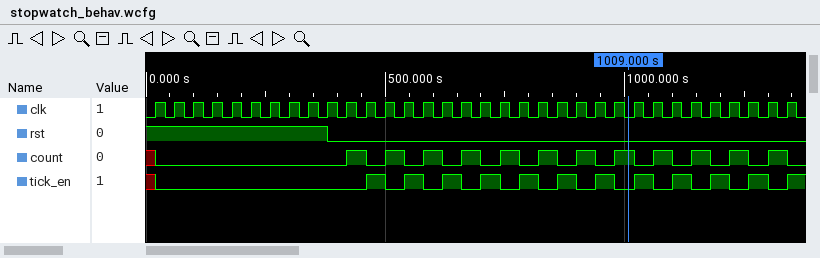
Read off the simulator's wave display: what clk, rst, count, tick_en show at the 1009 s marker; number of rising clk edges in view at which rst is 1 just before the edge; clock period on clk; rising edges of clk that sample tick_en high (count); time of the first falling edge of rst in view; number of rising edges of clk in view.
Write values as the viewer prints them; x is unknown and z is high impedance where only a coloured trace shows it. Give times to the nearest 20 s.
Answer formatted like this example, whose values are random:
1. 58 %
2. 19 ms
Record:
1. clk=0, rst=0, count=1, tick_en=0
2. 10
3. 40 s
4. 11
5. 380 s
6. 34
